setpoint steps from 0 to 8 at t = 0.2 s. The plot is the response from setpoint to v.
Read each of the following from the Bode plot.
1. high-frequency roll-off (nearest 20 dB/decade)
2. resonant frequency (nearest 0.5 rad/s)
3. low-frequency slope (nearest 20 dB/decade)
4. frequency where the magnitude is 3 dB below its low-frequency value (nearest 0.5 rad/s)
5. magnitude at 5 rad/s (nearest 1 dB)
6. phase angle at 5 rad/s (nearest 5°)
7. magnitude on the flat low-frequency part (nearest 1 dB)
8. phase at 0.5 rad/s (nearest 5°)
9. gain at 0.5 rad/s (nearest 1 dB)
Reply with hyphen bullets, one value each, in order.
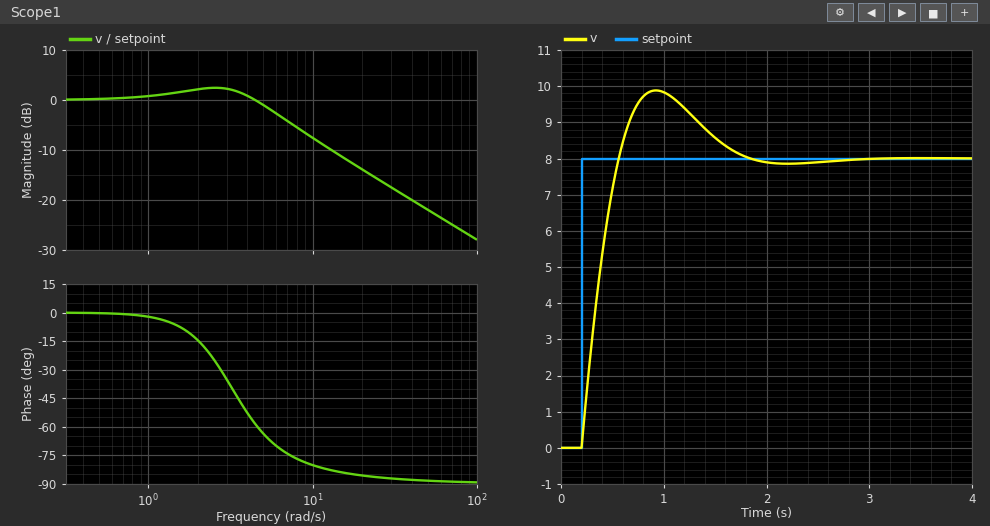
- -20 dB/decade
- 2.5 rad/s
- 0 dB/decade
- 6.0 rad/s
- -1 dB
- -65°
- 0 dB
- 0°
- 0 dB
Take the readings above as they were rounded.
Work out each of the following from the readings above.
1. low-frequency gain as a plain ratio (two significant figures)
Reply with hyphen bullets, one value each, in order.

- 1.0
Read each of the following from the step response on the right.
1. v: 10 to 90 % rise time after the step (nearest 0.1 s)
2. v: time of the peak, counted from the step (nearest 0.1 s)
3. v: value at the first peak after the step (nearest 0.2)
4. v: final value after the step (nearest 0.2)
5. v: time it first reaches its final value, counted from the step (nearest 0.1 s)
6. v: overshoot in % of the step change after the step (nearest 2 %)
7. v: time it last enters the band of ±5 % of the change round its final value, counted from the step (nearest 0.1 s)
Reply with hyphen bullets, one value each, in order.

- 0.3 s
- 0.7 s
- 9.8
- 8.0
- 0.4 s
- 24 %
- 1.4 s
